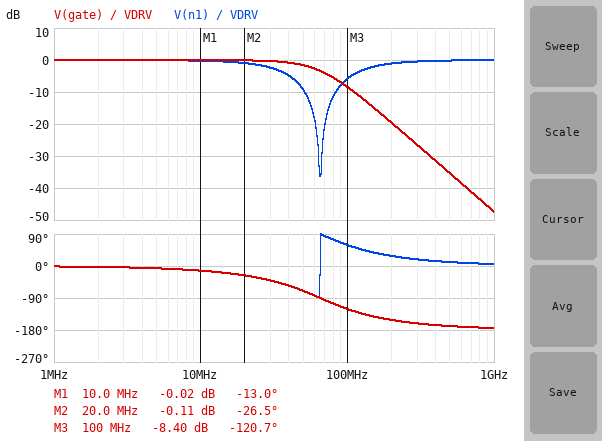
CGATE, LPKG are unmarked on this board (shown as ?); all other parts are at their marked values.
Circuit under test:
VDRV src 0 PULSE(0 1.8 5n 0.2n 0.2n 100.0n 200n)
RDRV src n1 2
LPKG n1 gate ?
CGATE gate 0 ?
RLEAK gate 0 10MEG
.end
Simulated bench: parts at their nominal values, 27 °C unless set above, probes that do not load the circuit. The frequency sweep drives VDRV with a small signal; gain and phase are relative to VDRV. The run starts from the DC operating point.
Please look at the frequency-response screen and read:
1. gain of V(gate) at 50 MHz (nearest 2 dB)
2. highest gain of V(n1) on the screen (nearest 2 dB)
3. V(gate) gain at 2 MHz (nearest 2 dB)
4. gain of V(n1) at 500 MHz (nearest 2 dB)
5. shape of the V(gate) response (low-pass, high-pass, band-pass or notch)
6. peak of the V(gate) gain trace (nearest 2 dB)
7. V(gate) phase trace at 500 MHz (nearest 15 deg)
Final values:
-2 dB
0 dB
0 dB
0 dB
low-pass
0 dB
-165 deg
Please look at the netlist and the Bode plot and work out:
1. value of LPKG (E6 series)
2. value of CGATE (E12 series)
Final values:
3.3 nH
1.8 nF
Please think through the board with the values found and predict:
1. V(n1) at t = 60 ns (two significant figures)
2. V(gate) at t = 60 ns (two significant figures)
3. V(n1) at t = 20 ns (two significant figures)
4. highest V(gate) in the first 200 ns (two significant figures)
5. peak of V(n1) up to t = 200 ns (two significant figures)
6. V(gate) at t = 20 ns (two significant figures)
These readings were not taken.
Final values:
1.8 V
1.8 V
1.8 V
1.9 V
1.8 V
1.8 V
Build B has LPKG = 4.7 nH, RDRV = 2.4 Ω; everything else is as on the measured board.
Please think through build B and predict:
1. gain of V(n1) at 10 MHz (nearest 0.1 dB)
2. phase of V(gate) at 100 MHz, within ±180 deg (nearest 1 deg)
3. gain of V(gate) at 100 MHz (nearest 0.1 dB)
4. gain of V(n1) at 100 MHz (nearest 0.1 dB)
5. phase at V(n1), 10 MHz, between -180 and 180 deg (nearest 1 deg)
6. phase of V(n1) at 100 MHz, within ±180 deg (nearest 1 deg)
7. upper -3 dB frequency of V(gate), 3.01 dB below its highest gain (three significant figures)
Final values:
-0.3 dB
-131 deg
-11.1 dB
-3.7 dB
-16 deg
49 deg
52.0 MHz
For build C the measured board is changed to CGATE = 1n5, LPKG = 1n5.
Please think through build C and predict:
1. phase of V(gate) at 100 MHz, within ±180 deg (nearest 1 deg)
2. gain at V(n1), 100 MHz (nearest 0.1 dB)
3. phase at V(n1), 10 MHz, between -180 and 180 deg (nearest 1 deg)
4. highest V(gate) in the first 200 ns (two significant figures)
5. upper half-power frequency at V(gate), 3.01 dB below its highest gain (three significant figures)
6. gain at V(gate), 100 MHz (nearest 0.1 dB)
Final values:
-87 deg
-24.6 dB
-11 deg
1.8 V
68.3 MHz
-5.5 dB
